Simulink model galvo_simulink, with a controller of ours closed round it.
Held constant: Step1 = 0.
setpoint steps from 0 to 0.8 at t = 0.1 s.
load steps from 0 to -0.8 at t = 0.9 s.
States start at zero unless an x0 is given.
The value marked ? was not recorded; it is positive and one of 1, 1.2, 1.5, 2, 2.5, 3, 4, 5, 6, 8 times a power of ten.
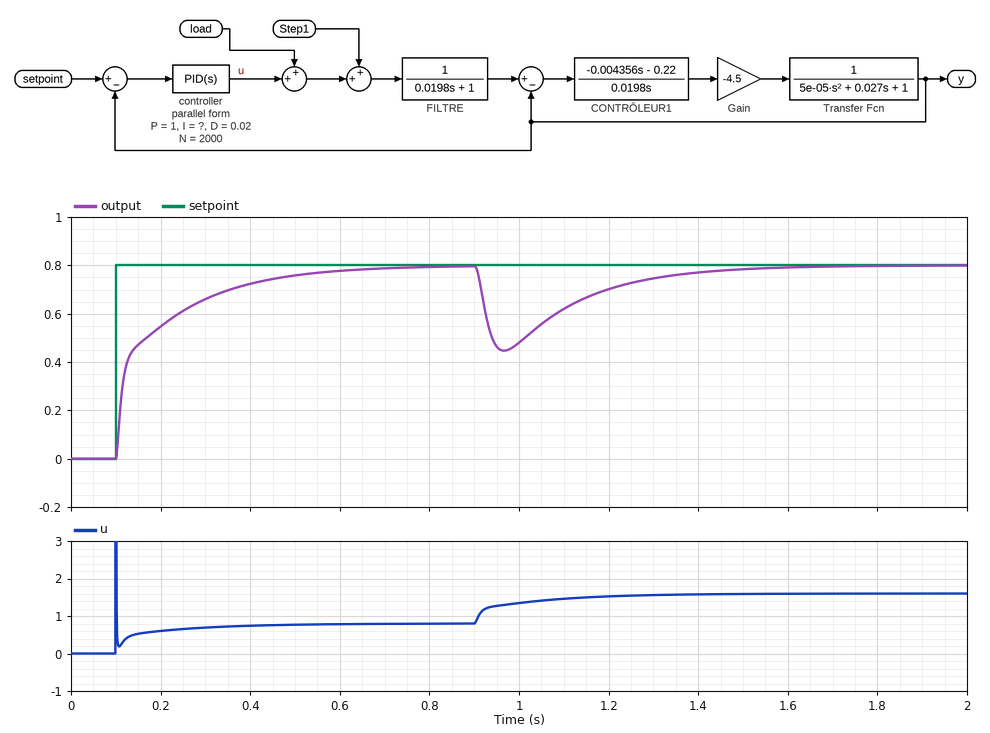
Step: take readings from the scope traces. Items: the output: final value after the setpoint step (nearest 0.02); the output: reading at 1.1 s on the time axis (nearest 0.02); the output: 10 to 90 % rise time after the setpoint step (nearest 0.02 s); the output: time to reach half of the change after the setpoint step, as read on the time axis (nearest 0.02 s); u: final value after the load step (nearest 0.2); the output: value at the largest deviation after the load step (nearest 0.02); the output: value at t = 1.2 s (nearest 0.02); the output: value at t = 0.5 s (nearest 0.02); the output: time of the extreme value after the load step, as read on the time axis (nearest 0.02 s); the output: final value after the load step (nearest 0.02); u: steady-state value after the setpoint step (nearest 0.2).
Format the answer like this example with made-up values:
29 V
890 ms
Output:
0.80
0.62
0.28 s
0.12 s
1.6
0.44
0.70
0.76
0.96 s
0.80
0.8
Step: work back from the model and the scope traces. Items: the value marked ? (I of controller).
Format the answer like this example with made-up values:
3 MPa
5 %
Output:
10
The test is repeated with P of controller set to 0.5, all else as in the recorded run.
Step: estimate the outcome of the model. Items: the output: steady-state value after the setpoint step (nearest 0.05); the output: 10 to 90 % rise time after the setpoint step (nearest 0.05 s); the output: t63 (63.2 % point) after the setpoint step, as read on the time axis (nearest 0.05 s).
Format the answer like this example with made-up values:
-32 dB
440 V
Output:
0.80
0.25 s
0.20 s
